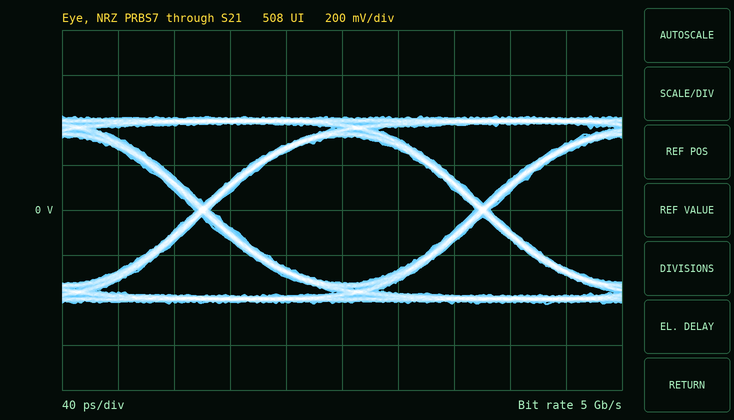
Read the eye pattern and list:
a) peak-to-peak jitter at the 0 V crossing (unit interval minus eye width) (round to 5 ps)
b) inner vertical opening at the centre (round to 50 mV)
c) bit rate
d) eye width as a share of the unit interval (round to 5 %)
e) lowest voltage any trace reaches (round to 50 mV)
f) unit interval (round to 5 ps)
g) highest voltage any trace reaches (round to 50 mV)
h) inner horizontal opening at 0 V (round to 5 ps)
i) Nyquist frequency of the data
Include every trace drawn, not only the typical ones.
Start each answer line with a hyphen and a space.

- 10 ps
- 650 mV
- 5 Gb/s
- 95 %
- -400 mV
- 200 ps
- 400 mV
- 190 ps
- 2.5 GHz
